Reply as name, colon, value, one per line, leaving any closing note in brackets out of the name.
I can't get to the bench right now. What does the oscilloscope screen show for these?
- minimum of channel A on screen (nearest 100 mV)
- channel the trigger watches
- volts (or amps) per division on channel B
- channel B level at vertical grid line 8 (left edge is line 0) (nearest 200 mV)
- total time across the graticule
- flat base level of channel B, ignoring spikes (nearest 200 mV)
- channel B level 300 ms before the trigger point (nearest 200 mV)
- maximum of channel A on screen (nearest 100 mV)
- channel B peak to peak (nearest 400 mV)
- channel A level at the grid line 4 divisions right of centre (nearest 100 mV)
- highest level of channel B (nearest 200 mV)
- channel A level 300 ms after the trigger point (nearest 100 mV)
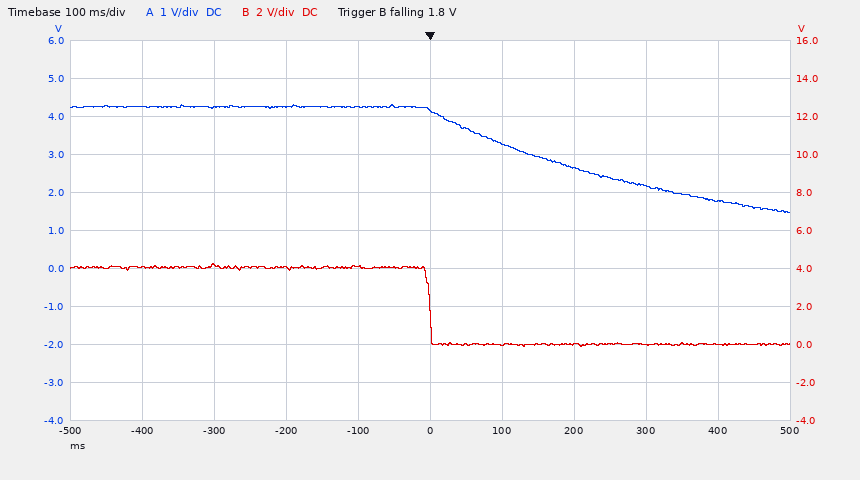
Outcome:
minimum of channel A on screen: 1.5 V
channel the trigger watches: channel B
volts (or amps) per division on channel B: 2 V
channel B level at vertical grid line 8 (left edge is line 0): 0.0 V
total time across the graticule: 1 s
flat base level of channel B, ignoring spikes: 0.0 V
channel B level 300 ms before the trigger point: 4.2 V
maximum of channel A on screen: 4.3 V
channel B peak to peak: 4.4 V
channel A level at the grid line 4 divisions right of centre: 1.8 V
highest level of channel B: 4.2 V
channel A level 300 ms after the trigger point: 2.2 V
